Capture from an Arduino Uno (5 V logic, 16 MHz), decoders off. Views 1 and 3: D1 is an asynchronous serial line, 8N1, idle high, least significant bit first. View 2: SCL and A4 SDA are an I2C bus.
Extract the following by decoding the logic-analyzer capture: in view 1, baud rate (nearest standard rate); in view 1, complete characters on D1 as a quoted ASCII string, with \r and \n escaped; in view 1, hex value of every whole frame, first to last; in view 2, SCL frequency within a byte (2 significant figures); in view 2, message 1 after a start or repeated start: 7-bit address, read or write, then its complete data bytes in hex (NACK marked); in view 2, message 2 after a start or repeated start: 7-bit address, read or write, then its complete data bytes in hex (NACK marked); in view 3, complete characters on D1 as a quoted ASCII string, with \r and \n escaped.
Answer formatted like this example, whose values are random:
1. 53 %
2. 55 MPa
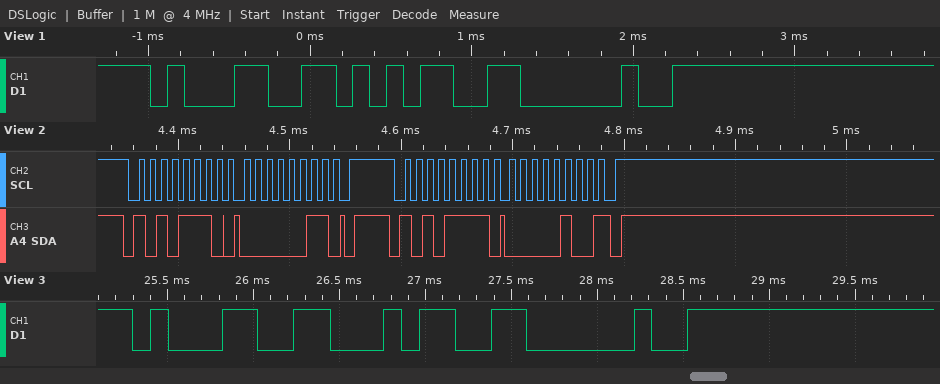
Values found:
1. 9600 baud
2. "15 "
3. 31 35 20
4. 100 kHz
5. 0x57 write: 03
6. 0x57 read: 04 NACK
7. "14 "
